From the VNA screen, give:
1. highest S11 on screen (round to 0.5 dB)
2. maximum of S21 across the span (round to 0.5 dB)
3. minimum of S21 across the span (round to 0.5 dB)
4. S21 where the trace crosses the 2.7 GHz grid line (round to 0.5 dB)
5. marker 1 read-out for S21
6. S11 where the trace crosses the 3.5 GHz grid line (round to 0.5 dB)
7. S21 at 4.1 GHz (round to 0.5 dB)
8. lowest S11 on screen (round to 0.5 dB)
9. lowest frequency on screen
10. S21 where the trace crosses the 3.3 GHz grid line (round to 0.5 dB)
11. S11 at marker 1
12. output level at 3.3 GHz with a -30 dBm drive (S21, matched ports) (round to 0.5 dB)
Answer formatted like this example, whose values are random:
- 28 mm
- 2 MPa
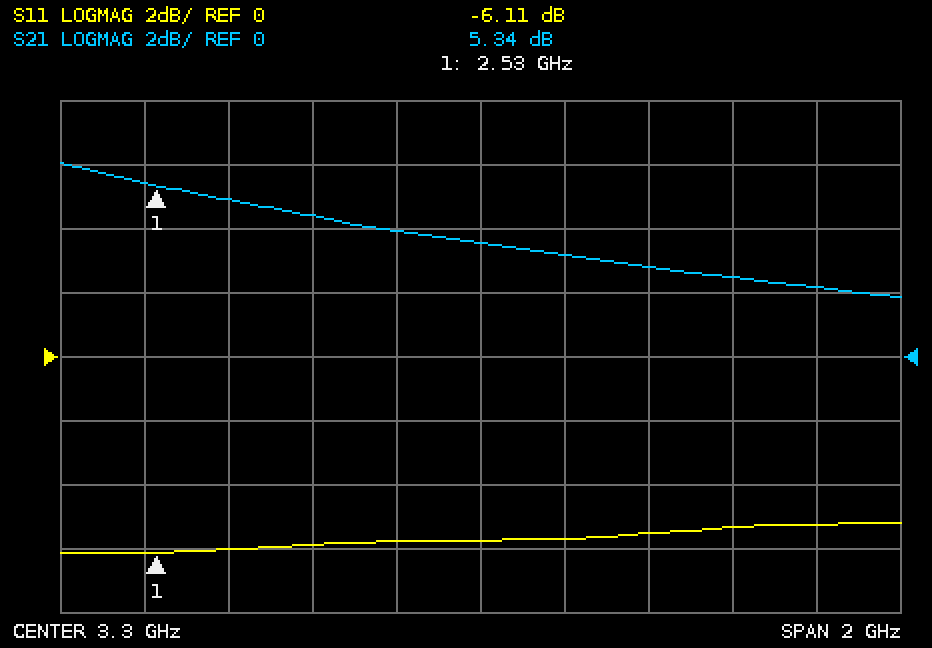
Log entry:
- -5.0 dB
- 6.0 dB
- 2.0 dB
- 5.0 dB
- 5.34 dB
- -5.5 dB
- 2.0 dB
- -6.0 dB
- 2.3 GHz
- 3.5 dB
- -6.11 dB
- -26.5 dBm
